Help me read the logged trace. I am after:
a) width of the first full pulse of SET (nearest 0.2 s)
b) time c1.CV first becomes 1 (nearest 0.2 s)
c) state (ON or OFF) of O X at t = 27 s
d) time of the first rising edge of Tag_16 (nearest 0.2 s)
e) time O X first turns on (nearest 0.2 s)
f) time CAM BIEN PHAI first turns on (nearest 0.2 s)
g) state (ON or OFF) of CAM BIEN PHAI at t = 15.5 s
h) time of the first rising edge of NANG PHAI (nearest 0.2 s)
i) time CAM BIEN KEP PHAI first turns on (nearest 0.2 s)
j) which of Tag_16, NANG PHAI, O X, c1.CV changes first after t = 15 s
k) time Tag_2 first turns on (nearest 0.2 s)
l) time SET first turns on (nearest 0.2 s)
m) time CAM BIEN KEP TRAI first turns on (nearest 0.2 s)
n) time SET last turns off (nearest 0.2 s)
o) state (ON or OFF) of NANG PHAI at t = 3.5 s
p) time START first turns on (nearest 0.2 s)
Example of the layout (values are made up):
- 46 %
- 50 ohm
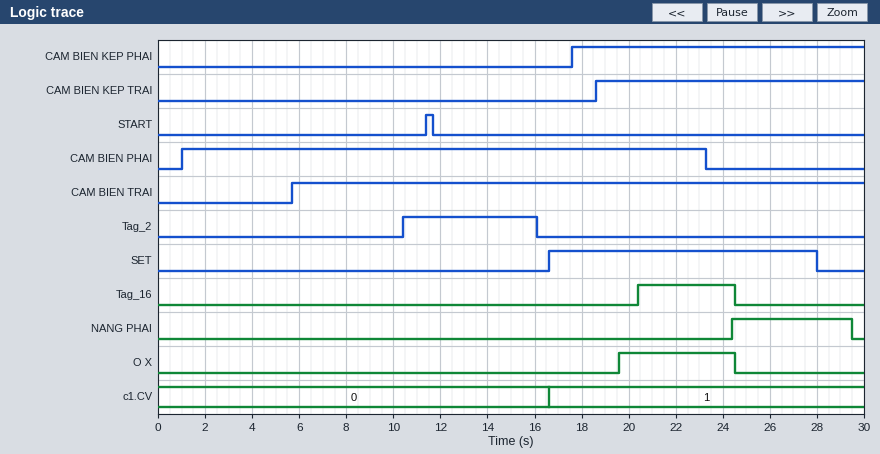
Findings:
- 11.4 s
- 16.6 s
- OFF
- 20.4 s
- 19.6 s
- 1.0 s
- ON
- 24.4 s
- 17.6 s
- c1.CV
- 10.4 s
- 16.6 s
- 18.6 s
- 28.0 s
- OFF
- 11.4 s
